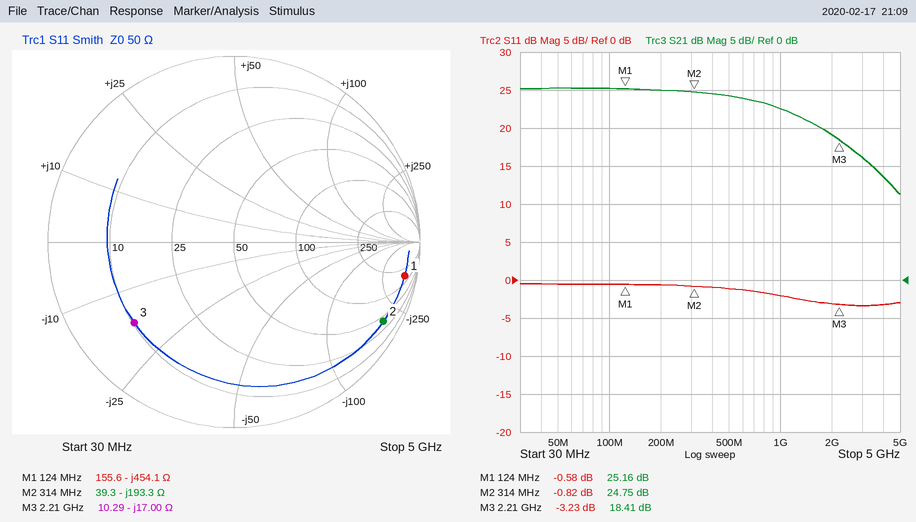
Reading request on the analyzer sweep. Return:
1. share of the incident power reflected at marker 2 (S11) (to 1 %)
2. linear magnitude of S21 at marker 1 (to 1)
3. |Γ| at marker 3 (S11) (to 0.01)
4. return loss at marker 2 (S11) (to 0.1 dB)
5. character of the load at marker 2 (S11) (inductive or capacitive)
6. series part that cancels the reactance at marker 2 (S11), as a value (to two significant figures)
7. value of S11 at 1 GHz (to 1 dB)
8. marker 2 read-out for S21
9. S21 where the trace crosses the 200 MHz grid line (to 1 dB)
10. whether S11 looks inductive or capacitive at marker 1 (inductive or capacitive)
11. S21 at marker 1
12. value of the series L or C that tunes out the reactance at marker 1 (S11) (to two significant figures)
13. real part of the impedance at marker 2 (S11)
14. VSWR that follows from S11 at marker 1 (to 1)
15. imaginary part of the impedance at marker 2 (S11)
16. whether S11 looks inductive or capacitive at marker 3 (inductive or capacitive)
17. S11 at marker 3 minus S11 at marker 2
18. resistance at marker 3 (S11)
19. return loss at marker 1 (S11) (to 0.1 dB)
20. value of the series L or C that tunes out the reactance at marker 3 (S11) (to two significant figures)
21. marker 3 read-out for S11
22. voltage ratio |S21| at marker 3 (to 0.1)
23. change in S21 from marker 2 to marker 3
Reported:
83 %
18
0.69
0.8 dB
capacitive
98 nH
-2 dB
24.75 dB
25 dB
capacitive
25.16 dB
580 nH
39.3 Ω
30
-193.3 Ω
capacitive
-2.41 dB
10.29 Ω
0.6 dB
1.2 nH
-3.23 dB
8.3
-6.34 dB
